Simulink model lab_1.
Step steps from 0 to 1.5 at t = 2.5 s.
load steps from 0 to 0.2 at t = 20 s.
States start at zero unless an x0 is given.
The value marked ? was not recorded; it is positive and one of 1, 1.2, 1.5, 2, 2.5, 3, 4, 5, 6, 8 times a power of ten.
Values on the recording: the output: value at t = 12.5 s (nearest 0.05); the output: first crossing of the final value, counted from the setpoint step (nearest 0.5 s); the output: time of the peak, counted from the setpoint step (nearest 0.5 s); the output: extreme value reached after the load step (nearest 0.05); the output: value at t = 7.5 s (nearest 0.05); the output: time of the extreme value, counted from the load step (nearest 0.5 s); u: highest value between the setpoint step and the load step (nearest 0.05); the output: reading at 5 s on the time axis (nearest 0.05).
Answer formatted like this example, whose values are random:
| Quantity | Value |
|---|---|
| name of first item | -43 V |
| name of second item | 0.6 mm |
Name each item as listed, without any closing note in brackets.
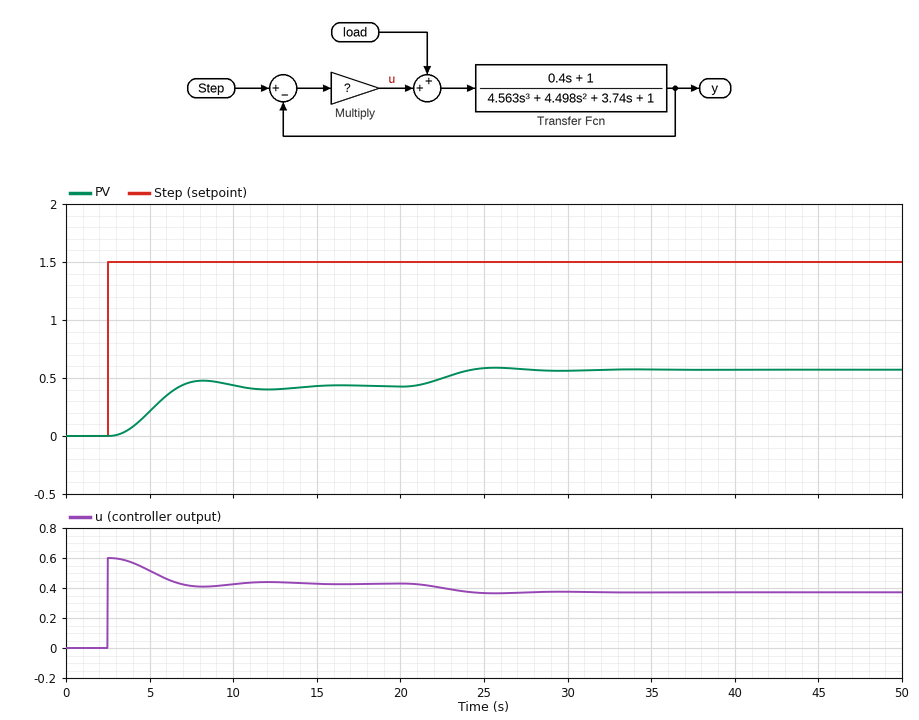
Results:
| Quantity | Value |
|---|---|
| the output: value at t = 12.5 s | 0.40 |
| the output: first crossing of the final value, counted from the setpoint step | 4.5 s |
| the output: time of the peak, counted from the setpoint step | 5.5 s |
| the output: extreme value reached after the load step | 0.60 |
| the output: value at t = 7.5 s | 0.45 |
| the output: time of the extreme value, counted from the load step | 5.5 s |
| u: highest value between the setpoint step and the load step | 0.60 |
| the output: reading at 5 s on the time axis | 0.20 |
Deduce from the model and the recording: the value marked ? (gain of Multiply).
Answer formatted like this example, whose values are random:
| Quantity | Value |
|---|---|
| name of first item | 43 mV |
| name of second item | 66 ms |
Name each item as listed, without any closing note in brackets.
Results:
| Quantity | Value |
|---|---|
| the value marked ? | 0.4 |
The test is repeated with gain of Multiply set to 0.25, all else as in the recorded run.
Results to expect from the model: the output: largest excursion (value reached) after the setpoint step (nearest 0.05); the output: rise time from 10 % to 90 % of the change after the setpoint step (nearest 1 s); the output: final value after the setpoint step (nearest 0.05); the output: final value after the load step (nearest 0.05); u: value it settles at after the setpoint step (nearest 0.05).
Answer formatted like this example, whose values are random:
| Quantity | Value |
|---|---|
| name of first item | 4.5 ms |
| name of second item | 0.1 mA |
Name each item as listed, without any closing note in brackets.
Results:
| Quantity | Value |
|---|---|
| the output: largest excursion (value reached) after the setpoint step | 0.30 |
| the output: rise time from 10 % to 90 % of the change after the setpoint step | 3 s |
| the output: final value after the setpoint step | 0.30 |
| the output: final value after the load step | 0.45 |
| u: value it settles at after the setpoint step | 0.30 |
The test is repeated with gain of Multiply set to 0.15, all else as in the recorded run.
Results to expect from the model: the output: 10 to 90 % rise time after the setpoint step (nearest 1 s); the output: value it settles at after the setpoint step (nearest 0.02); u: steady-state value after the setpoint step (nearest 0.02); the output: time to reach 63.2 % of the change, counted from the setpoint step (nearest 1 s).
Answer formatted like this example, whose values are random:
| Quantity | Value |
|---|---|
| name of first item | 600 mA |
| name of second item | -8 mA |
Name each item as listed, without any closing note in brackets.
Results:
| Quantity | Value |
|---|---|
| the output: 10 to 90 % rise time after the setpoint step | 3 s |
| the output: value it settles at after the setpoint step | 0.20 |
| u: steady-state value after the setpoint step | 0.20 |
| the output: time to reach 63.2 % of the change, counted from the setpoint step | 3 s |
